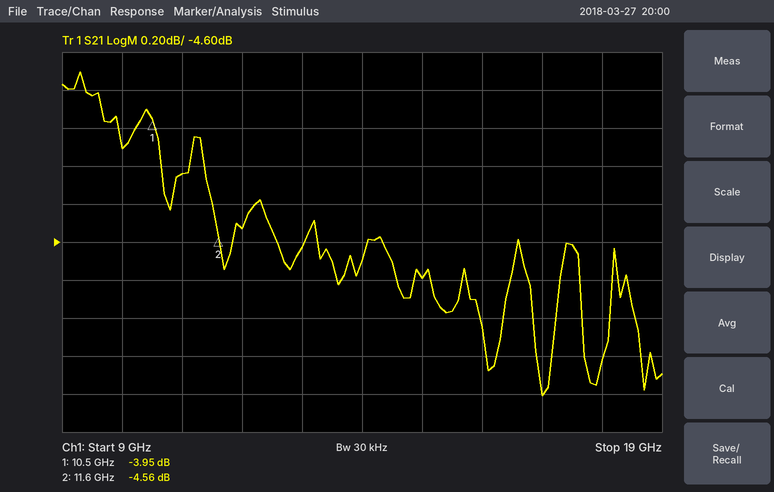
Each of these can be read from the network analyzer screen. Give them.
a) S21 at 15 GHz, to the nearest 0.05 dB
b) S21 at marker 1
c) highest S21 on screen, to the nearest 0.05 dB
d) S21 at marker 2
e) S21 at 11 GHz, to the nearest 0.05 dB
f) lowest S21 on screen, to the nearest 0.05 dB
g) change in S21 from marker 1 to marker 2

-4.80 dB
-3.95 dB
-3.70 dB
-4.56 dB
-4.25 dB
-5.40 dB
-0.61 dB
